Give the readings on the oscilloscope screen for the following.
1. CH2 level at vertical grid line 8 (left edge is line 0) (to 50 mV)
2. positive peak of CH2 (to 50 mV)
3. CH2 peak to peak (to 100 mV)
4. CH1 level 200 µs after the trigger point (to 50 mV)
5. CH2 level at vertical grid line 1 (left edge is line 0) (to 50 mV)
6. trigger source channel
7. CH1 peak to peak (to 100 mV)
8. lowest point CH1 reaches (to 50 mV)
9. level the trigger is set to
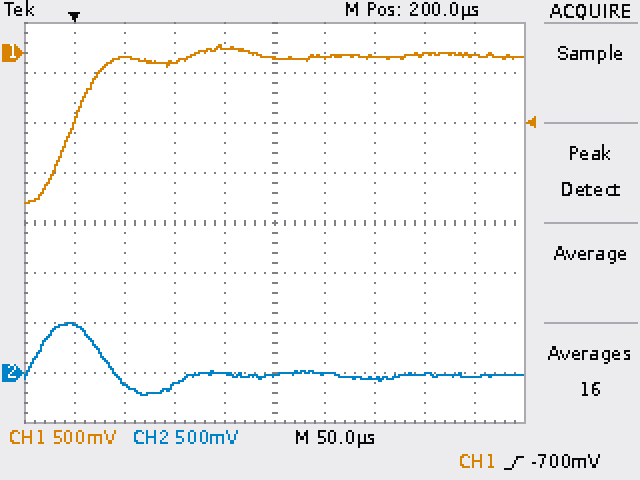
0 mV
500 mV
700 mV
-50 mV
500 mV
CH1
1.60 V
-1.50 V
-700 mV
